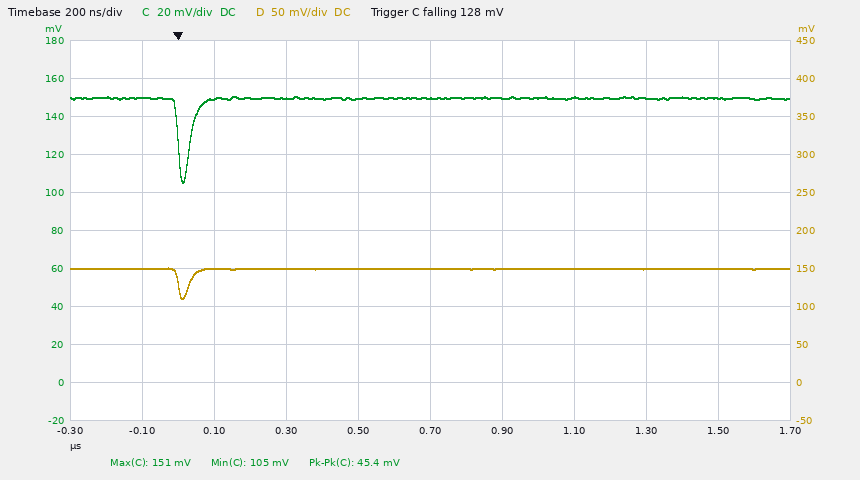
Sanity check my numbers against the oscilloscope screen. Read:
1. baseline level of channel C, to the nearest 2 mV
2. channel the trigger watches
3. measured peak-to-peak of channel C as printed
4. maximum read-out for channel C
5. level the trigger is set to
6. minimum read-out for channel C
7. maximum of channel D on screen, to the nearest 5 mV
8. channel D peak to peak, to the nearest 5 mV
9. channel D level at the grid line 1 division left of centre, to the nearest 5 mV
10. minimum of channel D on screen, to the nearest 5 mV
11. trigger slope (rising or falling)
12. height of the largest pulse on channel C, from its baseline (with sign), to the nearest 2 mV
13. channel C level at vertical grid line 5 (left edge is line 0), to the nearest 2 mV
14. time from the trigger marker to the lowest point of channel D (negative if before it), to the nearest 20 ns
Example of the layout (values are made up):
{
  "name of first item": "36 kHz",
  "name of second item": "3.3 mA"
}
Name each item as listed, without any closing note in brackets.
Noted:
{
  "baseline level of channel C, to the nearest 2 mV": "150 mV",
  "channel the trigger watches": "channel C",
  "measured peak-to-peak of channel C as printed": "45.4 mV",
  "maximum read-out for channel C": "151 mV",
  "level the trigger is set to": "128 mV",
  "minimum read-out for channel C": "105 mV",
  "maximum of channel D on screen, to the nearest 5 mV": "150 mV",
  "channel D peak to peak, to the nearest 5 mV": "40 mV",
  "channel D level at the grid line 1 division left of centre, to the nearest 5 mV": "150 mV",
  "minimum of channel D on screen, to the nearest 5 mV": "110 mV",
  "trigger slope": "falling",
  "height of the largest pulse on channel C, from its baseline (with sign), to the nearest 2 mV": "-44 mV",
  "channel C level at vertical grid line 5 (left edge is line 0), to the nearest 2 mV": "150 mV",
  "time from the trigger marker to the lowest point of channel D (negative if before it), to the nearest 20 ns": "+20 ns"
}
